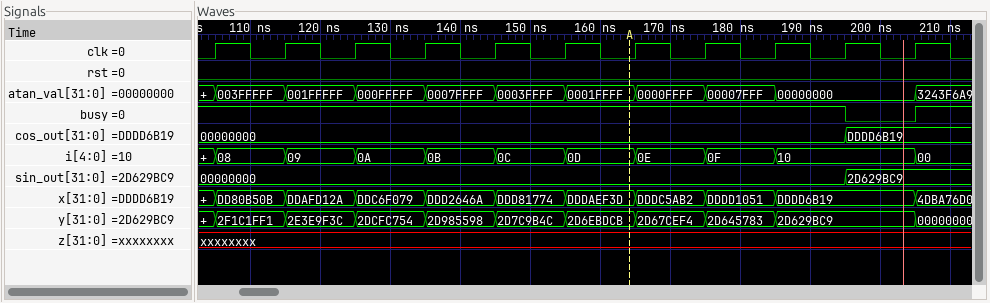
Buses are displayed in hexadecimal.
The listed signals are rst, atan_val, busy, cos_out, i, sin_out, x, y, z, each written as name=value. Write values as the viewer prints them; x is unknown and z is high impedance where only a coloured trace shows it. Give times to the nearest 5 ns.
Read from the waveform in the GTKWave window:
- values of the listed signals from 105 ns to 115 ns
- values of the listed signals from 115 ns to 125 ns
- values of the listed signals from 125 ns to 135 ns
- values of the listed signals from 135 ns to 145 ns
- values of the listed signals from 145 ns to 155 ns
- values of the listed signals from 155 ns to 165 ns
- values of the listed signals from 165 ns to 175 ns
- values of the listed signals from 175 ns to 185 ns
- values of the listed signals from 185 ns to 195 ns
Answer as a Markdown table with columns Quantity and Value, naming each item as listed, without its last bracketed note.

| Quantity | Value |
|---|---|
| values of the listed signals from 105 ns to 115 ns | rst=0, atan_val=003FFFFF, busy=1, cos_out=00000000, i=08, sin_out=00000000, x=DD80B50B, y=2F1C1FF1, z=xxxxxxxx |
| values of the listed signals from 115 ns to 125 ns | rst=0, atan_val=001FFFFF, busy=1, cos_out=00000000, i=09, sin_out=00000000, x=DDAFD12A, y=2E3E9F3C, z=xxxxxxxx |
| values of the listed signals from 125 ns to 135 ns | rst=0, atan_val=000FFFFF, busy=1, cos_out=00000000, i=0A, sin_out=00000000, x=DDC6F079, y=2DCFC754, z=xxxxxxxx |
| values of the listed signals from 135 ns to 145 ns | rst=0, atan_val=0007FFFF, busy=1, cos_out=00000000, i=0B, sin_out=00000000, x=DDD2646A, y=2D985598, z=xxxxxxxx |
| values of the listed signals from 145 ns to 155 ns | rst=0, atan_val=0003FFFF, busy=1, cos_out=00000000, i=0C, sin_out=00000000, x=DDD81774, y=2D7C9B4C, z=xxxxxxxx |
| values of the listed signals from 155 ns to 165 ns | rst=0, atan_val=0001FFFF, busy=1, cos_out=00000000, i=0D, sin_out=00000000, x=DDDAEF3D, y=2D6EBDCB, z=xxxxxxxx |
| values of the listed signals from 165 ns to 175 ns | rst=0, atan_val=0000FFFF, busy=1, cos_out=00000000, i=0E, sin_out=00000000, x=DDDC5AB2, y=2D67CEF4, z=xxxxxxxx |
| values of the listed signals from 175 ns to 185 ns | rst=0, atan_val=00007FFF, busy=1, cos_out=00000000, i=0F, sin_out=00000000, x=DDDD1051, y=2D645783, z=xxxxxxxx |
| values of the listed signals from 185 ns to 195 ns | rst=0, atan_val=00000000, busy=1, cos_out=00000000, i=10, sin_out=00000000, x=DDDD6B19, y=2D629BC9, z=xxxxxxxx |
